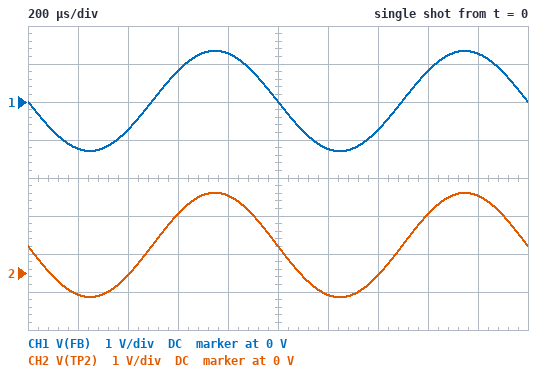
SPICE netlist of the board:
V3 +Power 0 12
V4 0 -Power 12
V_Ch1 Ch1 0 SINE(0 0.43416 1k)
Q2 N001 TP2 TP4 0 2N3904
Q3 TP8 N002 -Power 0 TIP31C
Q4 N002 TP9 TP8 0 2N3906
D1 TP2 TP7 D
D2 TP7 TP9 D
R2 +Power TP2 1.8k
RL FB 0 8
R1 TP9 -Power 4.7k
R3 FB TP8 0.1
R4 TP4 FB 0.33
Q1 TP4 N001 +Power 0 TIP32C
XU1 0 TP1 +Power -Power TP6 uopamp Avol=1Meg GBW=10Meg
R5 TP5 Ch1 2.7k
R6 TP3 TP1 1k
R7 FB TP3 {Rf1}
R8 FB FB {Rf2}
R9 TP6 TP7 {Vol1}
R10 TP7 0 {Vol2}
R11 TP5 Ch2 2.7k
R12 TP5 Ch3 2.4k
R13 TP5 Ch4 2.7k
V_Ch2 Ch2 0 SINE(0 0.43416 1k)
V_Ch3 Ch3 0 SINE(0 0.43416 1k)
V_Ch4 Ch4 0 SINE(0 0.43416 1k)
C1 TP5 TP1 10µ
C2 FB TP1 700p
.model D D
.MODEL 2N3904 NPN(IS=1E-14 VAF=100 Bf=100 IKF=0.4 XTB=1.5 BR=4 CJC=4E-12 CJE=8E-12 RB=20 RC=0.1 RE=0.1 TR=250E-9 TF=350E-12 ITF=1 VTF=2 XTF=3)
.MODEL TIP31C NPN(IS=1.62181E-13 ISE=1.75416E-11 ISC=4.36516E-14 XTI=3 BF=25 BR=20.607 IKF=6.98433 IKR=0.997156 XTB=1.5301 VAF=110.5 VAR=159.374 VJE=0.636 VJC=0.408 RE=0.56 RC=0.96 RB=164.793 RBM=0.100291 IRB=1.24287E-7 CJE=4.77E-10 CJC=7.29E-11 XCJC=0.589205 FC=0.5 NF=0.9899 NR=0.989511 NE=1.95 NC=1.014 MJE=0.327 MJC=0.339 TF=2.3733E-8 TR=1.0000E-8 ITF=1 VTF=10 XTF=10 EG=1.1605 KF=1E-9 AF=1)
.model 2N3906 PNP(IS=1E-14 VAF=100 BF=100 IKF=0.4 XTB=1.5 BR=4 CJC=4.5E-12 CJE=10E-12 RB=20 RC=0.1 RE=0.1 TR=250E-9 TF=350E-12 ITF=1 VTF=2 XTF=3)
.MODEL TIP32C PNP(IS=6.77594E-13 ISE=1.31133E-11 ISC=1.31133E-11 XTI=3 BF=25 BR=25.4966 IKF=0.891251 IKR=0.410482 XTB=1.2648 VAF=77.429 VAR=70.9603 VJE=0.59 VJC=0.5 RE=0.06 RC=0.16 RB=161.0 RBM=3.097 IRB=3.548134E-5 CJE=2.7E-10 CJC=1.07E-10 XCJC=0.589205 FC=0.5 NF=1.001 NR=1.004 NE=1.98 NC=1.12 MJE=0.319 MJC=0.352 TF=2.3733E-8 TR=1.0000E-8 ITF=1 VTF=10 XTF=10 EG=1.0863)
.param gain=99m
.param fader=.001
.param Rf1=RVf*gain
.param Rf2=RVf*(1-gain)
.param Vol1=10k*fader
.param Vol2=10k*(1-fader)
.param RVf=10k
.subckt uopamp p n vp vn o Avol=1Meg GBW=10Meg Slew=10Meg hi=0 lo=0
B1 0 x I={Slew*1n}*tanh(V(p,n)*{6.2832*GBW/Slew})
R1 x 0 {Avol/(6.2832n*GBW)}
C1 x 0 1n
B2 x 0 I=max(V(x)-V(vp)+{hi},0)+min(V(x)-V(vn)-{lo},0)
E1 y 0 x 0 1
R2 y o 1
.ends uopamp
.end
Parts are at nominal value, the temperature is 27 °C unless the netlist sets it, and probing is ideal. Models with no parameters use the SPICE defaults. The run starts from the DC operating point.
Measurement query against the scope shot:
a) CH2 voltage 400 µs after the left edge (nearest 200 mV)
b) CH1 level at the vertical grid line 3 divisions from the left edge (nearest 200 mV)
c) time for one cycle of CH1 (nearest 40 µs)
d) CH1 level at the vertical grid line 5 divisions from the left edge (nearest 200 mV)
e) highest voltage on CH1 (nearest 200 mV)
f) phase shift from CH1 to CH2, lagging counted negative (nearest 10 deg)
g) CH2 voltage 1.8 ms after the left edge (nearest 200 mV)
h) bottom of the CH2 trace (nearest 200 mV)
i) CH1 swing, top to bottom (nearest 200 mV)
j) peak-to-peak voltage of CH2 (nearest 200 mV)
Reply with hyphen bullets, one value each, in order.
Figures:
- 0 V
- 800 mV
- 1.00 ms
- 0 V
- 1.4 V
- 0 deg
- 2.0 V
- -600 mV
- 2.6 V
- 2.8 V
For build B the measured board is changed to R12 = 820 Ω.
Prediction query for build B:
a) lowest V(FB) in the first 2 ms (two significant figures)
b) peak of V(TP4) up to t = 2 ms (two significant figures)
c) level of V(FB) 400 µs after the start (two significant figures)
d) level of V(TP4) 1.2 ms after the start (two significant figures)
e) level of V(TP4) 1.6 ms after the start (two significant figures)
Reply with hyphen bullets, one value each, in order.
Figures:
- -2.0 V
- 2.2 V
- -1.1 V
- -1.9 V
- 1.3 V
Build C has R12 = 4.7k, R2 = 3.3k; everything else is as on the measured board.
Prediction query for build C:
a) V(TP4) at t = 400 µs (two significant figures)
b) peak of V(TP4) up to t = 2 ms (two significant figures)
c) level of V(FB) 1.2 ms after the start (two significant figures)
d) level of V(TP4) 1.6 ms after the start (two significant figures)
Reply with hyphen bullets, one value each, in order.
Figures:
- -630 mV
- 1.2 V
- -1.1 V
- 740 mV
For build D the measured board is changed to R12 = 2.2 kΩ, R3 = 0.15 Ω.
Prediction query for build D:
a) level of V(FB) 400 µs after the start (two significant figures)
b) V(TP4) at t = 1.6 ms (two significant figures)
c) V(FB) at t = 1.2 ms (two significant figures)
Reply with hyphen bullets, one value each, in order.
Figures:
- -750 mV
- 880 mV
- -1.3 V
